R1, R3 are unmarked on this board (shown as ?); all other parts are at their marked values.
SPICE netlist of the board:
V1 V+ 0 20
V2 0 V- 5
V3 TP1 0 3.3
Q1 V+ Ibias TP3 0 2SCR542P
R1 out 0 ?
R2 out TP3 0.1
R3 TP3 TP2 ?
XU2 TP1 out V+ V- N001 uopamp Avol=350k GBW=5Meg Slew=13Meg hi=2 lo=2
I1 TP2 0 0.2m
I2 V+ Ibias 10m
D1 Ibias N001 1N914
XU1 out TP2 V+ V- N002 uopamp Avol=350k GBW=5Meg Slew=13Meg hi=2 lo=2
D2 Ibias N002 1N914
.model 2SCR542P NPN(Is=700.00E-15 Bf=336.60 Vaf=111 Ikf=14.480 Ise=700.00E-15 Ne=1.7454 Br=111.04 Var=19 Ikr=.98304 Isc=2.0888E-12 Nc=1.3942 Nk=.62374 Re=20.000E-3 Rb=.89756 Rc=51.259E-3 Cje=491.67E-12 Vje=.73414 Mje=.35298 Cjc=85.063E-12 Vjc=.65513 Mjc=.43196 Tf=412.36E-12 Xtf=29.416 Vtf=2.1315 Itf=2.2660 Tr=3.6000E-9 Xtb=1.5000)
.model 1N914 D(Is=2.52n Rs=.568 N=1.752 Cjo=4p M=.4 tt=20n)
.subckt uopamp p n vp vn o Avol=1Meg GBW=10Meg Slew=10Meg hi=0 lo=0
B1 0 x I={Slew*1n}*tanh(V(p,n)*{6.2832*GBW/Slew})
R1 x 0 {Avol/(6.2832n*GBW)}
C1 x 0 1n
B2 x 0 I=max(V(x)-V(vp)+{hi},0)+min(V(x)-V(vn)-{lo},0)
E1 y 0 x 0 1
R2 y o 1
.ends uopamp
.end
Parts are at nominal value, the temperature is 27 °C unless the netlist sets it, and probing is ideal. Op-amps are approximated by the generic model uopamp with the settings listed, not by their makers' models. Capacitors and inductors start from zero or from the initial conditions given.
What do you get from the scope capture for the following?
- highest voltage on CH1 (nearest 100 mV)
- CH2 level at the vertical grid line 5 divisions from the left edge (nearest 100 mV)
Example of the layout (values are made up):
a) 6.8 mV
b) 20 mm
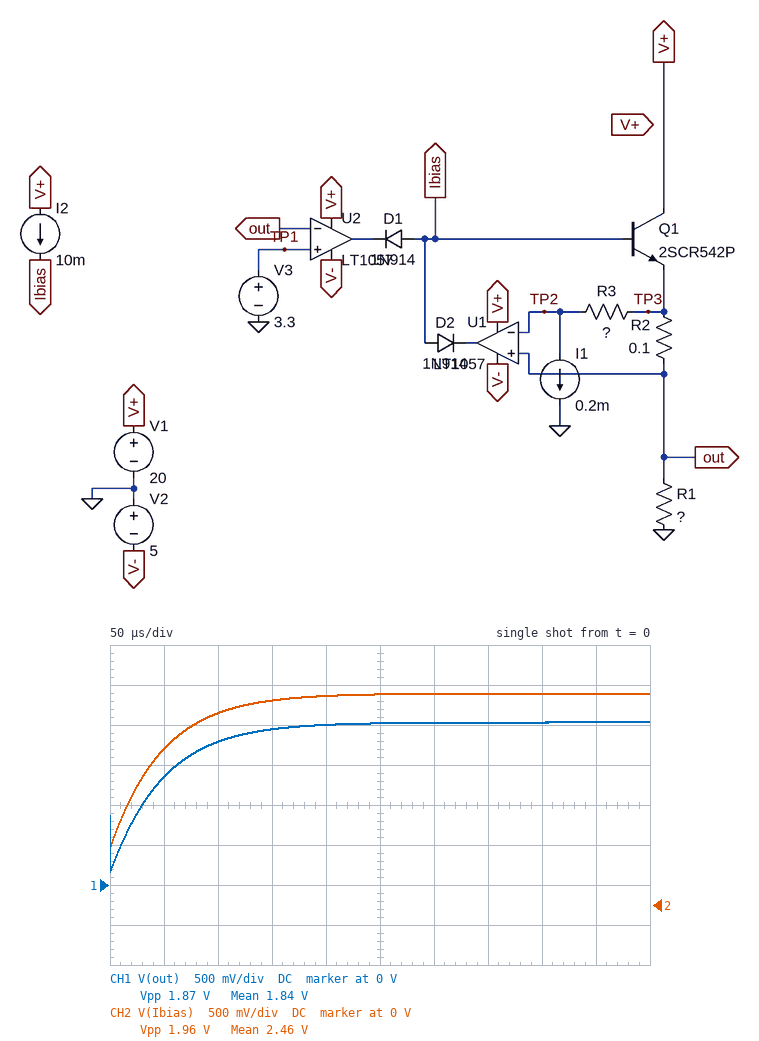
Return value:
a) 2.0 V
b) 2.6 V
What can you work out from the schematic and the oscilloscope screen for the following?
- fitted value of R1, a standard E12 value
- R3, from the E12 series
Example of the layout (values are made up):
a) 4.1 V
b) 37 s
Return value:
a) 150 Ω
b) 6.8 Ω
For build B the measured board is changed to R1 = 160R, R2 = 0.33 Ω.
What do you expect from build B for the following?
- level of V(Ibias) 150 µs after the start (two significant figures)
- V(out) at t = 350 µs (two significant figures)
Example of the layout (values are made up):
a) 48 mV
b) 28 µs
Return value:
a) 1.2 V
b) 660 mV
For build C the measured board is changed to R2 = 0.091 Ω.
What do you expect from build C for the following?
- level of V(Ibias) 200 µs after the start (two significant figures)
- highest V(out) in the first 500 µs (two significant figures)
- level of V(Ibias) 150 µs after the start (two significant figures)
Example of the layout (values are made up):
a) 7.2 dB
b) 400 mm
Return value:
a) 2.8 V
b) 2.2 V
c) 2.7 V
